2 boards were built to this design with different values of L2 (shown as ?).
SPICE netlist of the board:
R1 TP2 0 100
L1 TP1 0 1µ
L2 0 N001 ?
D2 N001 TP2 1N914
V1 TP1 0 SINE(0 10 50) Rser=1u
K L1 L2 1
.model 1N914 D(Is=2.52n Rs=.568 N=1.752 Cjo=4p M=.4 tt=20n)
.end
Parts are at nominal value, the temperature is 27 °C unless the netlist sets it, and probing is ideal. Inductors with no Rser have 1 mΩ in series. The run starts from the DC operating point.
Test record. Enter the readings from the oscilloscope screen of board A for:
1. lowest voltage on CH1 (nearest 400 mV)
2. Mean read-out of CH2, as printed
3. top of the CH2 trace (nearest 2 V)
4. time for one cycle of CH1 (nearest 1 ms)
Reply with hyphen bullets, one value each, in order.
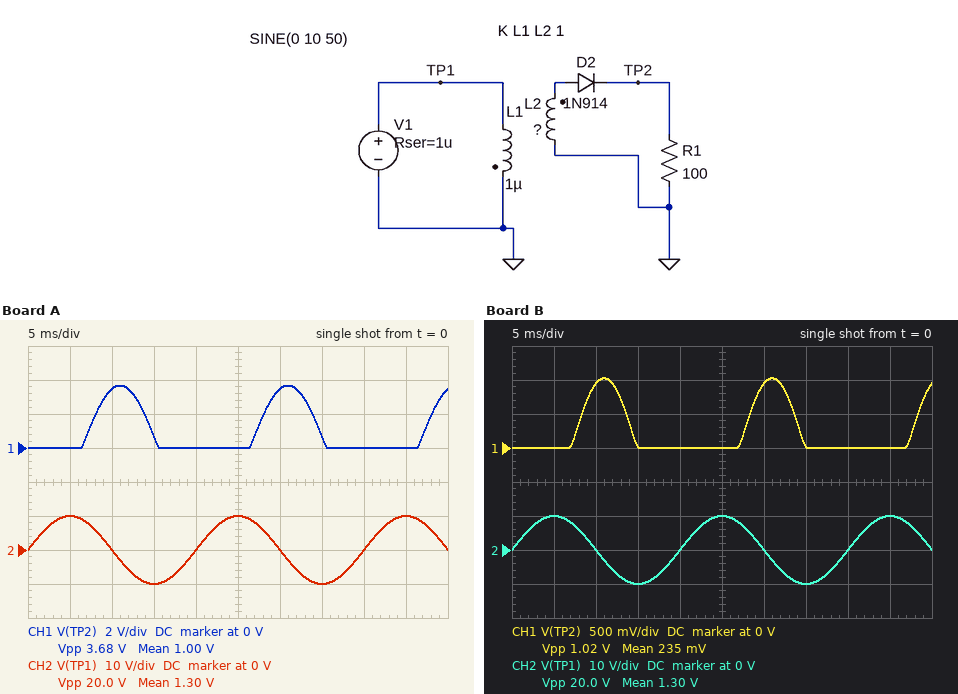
- 0 V
- 1.30 V
- 10 V
- 20 ms
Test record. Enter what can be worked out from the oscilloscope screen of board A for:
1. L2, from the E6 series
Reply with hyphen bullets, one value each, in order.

- 2.2 µH
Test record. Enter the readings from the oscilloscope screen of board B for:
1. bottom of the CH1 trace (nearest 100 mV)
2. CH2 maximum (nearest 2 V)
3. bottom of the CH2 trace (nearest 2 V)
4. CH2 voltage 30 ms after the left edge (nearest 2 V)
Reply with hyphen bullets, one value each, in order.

- 0 V
- 10 V
- -10 V
- 0 V
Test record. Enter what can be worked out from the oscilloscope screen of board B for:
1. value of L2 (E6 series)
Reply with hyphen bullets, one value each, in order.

- 330 nH
